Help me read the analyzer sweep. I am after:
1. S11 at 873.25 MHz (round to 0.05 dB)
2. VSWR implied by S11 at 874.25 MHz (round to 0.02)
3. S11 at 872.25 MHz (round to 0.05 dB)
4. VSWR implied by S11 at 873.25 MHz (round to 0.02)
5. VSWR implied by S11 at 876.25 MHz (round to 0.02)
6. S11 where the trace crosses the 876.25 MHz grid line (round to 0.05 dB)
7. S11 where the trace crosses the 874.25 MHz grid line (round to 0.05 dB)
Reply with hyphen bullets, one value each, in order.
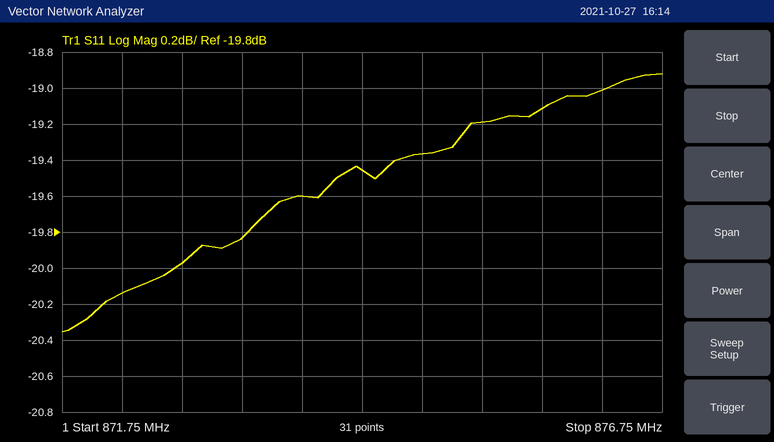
- -19.85 dB
- 1.24
- -20.15 dB
- 1.22
- 1.26
- -19.00 dB
- -19.45 dB
